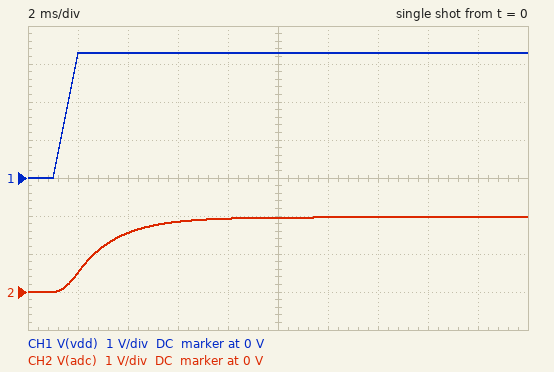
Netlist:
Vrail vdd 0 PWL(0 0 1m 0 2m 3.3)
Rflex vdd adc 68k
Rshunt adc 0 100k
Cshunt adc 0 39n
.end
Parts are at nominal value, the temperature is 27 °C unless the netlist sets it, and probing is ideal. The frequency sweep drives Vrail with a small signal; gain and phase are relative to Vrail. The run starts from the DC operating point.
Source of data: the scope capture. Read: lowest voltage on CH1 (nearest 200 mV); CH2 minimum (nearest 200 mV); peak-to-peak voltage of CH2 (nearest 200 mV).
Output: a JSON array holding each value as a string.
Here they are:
["0 V", "0 V", "2.0 V"]
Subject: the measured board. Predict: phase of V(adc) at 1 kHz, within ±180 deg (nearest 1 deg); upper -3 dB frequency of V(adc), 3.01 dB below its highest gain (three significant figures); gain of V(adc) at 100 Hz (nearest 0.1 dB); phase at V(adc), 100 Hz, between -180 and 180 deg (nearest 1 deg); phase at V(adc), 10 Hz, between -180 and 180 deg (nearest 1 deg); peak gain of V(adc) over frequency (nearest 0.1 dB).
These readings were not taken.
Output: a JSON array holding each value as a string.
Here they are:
["-84 deg", "101 Hz", "-7.5 dB", "-45 deg", "-6 deg", "-4.5 dB"]
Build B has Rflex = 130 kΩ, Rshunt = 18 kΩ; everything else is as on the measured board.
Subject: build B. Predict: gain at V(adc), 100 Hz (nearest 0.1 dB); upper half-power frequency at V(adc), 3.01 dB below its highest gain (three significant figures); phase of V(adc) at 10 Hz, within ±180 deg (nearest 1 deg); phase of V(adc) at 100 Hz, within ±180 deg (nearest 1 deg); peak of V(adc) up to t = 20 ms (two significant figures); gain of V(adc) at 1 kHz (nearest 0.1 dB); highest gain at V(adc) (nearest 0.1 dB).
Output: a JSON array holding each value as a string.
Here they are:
["-18.9 dB", "258 Hz", "-2 deg", "-21 deg", "400 mV", "-30.3 dB", "-18.3 dB"]
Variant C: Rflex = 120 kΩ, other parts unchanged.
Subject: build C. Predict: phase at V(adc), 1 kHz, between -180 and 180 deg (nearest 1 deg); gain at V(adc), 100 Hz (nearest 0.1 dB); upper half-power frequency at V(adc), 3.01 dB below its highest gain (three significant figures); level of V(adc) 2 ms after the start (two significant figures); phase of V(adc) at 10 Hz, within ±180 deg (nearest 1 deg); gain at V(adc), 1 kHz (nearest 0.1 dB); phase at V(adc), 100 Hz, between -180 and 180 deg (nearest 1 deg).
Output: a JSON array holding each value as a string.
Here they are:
["-86 deg", "-11.3 dB", "74.8 Hz", "300 mV", "-8 deg", "-29.4 dB", "-53 deg"]
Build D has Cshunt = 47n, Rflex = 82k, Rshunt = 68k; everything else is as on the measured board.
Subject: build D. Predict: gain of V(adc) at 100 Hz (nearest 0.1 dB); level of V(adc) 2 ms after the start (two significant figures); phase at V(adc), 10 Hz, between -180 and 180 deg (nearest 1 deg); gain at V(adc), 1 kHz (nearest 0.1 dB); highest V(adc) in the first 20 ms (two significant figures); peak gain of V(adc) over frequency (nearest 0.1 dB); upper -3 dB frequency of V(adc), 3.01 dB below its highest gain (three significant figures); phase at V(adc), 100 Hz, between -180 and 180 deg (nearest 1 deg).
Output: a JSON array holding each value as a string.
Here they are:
["-10.3 dB", "360 mV", "-6 deg", "-27.7 dB", "1.5 V", "-6.9 dB", "91.1 Hz", "-48 deg"]
